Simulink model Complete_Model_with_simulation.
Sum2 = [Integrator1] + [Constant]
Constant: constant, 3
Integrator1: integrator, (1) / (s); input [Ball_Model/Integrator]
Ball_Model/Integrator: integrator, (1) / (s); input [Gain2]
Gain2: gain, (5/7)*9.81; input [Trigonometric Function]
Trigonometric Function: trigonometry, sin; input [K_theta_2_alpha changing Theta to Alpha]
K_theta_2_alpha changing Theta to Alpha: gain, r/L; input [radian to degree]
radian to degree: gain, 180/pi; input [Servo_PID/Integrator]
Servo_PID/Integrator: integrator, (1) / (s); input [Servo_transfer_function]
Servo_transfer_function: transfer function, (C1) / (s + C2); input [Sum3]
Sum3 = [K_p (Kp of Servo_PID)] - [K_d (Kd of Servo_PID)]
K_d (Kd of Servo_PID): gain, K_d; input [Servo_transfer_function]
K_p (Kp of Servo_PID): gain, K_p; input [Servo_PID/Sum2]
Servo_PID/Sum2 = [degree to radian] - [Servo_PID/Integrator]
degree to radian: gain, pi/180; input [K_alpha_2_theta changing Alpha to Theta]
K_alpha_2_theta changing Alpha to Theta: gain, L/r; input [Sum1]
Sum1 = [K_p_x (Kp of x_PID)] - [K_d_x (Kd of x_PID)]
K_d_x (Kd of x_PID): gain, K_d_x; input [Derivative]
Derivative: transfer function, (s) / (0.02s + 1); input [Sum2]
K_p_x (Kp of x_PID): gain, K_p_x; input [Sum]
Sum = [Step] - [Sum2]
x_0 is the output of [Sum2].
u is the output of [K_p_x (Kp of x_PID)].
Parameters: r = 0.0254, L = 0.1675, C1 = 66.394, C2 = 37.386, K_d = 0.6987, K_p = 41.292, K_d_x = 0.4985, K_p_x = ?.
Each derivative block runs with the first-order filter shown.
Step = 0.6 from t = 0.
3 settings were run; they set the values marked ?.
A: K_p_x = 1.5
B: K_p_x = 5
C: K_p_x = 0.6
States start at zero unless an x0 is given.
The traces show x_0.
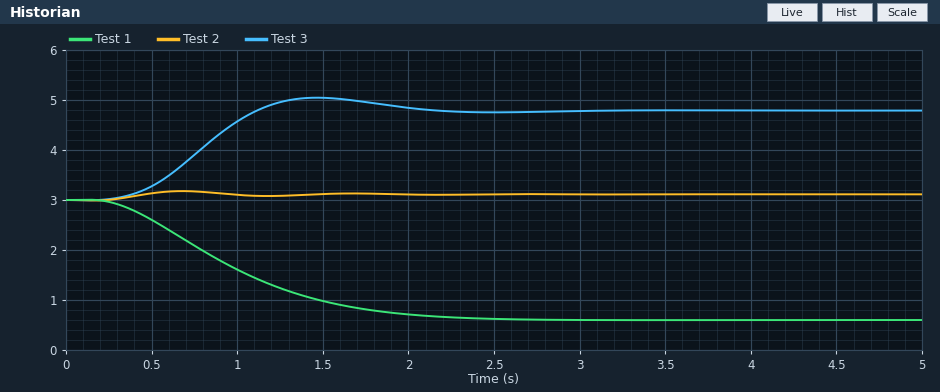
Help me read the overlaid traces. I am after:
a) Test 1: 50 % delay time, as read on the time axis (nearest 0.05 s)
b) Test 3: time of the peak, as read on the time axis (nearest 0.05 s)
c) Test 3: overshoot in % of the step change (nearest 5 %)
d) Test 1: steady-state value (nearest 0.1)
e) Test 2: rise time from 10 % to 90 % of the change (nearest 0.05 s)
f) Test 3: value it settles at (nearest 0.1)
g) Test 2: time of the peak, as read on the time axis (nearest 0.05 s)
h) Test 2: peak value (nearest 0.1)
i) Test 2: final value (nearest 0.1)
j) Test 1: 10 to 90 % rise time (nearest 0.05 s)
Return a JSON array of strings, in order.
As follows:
["0.90 s", "1.45 s", "15 %", "0.6", "0.15 s", "4.8", "0.70 s", "3.2", "3.1", "1.30 s"]
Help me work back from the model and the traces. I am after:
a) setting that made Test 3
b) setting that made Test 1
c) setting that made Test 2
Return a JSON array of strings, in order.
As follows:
["A", "C", "B"]
